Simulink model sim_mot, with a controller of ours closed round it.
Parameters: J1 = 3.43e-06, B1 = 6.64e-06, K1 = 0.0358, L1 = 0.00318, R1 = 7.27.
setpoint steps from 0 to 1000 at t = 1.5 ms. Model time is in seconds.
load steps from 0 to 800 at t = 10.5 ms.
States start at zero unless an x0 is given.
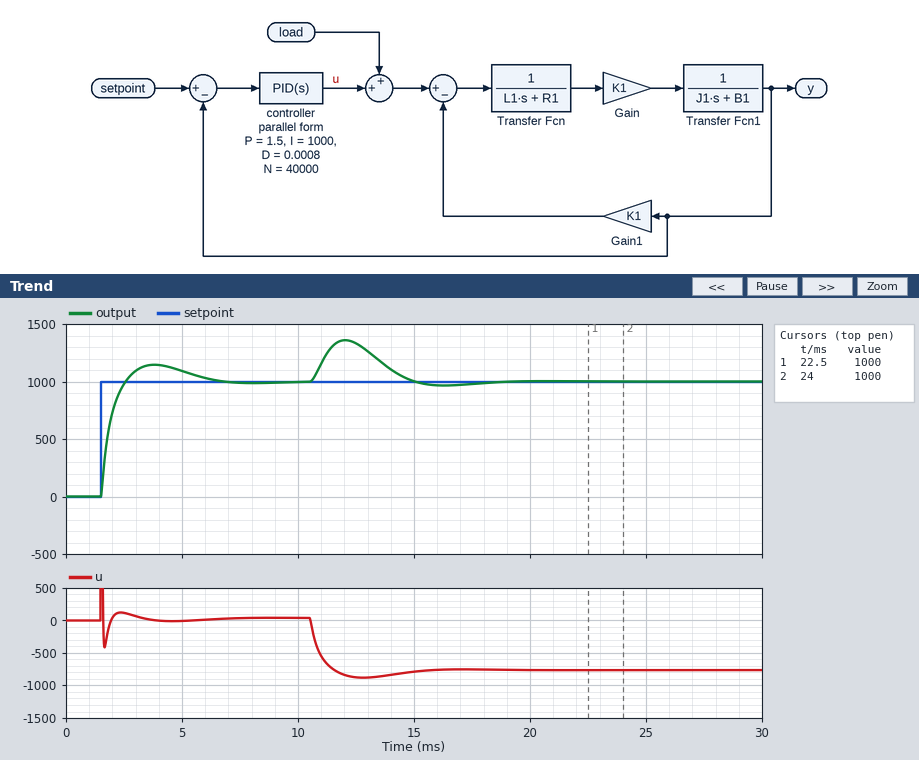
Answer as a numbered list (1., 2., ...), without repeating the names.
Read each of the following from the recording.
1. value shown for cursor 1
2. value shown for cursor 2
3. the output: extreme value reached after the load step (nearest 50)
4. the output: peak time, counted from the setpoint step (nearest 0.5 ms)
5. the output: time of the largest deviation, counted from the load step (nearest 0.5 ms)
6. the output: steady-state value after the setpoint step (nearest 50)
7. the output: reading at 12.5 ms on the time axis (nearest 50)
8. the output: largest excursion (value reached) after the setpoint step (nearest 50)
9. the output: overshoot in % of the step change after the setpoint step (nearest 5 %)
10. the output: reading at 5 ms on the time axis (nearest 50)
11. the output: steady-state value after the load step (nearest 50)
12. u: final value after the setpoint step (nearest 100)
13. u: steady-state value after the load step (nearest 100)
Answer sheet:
1. 1000
2. 1000
3. 1350
4. 2.5 ms
5. 1.5 ms
6. 1000
7. 1350
8. 1150
9. 15 %
10. 1100
11. 1000
12. 0
13. -800
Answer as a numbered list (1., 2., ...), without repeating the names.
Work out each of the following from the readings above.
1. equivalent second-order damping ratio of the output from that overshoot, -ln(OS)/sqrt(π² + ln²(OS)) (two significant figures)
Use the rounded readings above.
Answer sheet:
1. 0.52
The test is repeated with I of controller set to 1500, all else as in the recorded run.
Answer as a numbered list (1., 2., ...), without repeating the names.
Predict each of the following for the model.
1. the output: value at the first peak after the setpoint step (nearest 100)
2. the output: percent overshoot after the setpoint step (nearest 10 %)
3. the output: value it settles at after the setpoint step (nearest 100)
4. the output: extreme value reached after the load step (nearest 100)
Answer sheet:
1. 1200
2. 20 %
3. 1000
4. 1300
